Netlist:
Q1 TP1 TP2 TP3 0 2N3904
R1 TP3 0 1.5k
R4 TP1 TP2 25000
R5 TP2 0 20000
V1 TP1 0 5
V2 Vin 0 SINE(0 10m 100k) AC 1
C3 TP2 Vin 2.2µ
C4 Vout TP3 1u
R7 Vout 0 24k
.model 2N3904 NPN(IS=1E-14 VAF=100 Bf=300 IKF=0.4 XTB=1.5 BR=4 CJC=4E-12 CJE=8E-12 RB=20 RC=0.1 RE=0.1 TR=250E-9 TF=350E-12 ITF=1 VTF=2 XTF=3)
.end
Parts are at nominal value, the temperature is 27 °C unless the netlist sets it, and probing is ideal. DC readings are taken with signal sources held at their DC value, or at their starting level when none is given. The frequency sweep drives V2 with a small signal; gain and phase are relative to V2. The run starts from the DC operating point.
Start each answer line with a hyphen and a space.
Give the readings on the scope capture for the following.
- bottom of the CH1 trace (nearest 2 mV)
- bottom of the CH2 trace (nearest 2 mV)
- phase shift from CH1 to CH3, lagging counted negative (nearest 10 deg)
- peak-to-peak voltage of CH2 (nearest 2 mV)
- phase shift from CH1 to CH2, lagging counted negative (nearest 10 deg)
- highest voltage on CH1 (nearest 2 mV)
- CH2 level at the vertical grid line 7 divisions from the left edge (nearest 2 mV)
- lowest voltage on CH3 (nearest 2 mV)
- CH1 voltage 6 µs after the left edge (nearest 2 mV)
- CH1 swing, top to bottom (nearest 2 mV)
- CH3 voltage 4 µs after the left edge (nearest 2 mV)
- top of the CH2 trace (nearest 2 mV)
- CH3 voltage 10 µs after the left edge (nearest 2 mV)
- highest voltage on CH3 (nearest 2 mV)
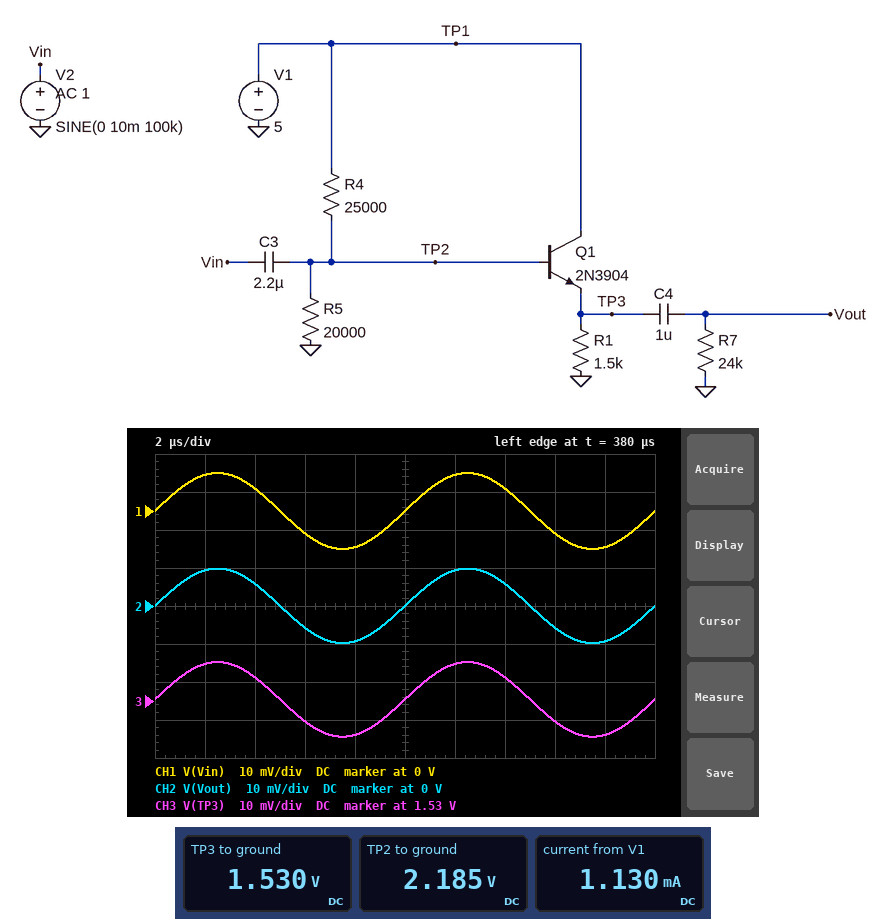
- -10 mV
- -10 mV
- 0 deg
- 20 mV
- 0 deg
- 10 mV
- 6 mV
- 1.520 V
- -6 mV
- 20 mV
- 1.536 V
- 10 mV
- 1.530 V
- 1.540 V
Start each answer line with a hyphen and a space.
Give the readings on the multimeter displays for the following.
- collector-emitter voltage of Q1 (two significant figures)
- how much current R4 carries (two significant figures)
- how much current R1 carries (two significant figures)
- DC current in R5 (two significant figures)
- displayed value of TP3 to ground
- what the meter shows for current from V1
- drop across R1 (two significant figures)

- 3.5 V
- 110 µA
- 1.0 mA
- 110 µA
- 1.530 V
- 1.130 mA
- 1.5 V
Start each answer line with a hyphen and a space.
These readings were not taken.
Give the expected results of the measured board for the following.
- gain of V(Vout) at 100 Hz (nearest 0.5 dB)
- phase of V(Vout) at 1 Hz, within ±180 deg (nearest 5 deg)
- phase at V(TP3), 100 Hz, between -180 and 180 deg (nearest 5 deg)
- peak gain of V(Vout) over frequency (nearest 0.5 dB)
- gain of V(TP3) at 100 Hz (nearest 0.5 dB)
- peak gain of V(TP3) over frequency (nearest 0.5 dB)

- 0 dB
- 165 deg
- 5 deg
- 0 dB
- 0 dB
- 0 dB
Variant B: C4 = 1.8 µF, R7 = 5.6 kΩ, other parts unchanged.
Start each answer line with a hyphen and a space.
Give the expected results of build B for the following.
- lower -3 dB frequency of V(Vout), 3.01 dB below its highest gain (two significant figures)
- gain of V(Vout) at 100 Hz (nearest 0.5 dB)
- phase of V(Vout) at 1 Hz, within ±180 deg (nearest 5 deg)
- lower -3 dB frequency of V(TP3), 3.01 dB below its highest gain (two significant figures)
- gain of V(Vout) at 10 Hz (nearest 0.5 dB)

- 18 Hz
- -0.5 dB
- 170 deg
- 6.6 Hz
- -7.0 dB
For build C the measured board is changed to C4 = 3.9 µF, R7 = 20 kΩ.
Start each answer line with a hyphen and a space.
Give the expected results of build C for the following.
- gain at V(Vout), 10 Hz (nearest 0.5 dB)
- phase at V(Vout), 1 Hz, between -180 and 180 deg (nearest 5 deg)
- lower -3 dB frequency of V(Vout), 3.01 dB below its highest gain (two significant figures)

- -2.0 dB
- 145 deg
- 7.2 Hz
